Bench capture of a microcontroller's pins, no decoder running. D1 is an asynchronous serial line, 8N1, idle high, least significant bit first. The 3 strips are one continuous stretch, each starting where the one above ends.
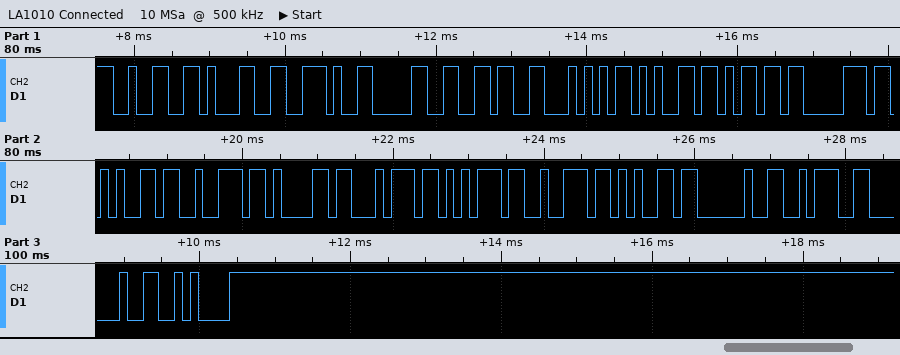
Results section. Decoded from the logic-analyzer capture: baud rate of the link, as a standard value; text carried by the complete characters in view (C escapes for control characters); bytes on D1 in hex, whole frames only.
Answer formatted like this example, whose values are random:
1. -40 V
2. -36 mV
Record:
1. 9600 baud
2. "21.06Temperature : \n"
3. 0x32 0x31 0x2E 0x30 0x36 0x54 0x65 0x6D 0x70 0x65 0x72 0x61 0x74 0x75 0x72 0x65 0x20 0x3A 0x20 0x0A
